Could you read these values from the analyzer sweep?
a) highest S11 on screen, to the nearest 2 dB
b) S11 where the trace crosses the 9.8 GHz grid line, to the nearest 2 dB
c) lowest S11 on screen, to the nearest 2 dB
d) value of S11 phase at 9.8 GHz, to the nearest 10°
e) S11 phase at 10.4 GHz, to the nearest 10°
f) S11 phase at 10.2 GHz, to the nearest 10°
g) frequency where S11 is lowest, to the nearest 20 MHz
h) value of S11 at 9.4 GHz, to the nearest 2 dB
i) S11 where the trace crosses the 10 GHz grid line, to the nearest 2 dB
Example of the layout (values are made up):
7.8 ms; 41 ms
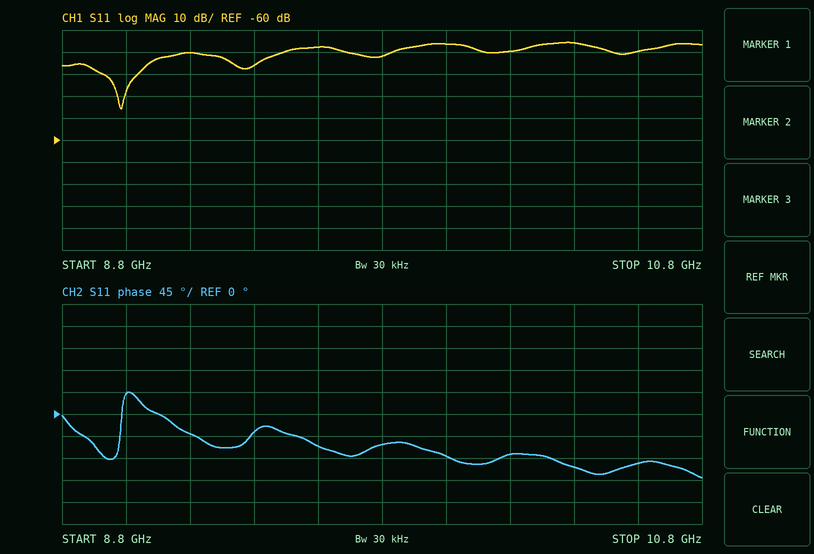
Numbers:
-16 dB; -22 dB; -46 dB; -60°; -110°; -80°; 8.98 GHz; -26 dB; -16 dB
